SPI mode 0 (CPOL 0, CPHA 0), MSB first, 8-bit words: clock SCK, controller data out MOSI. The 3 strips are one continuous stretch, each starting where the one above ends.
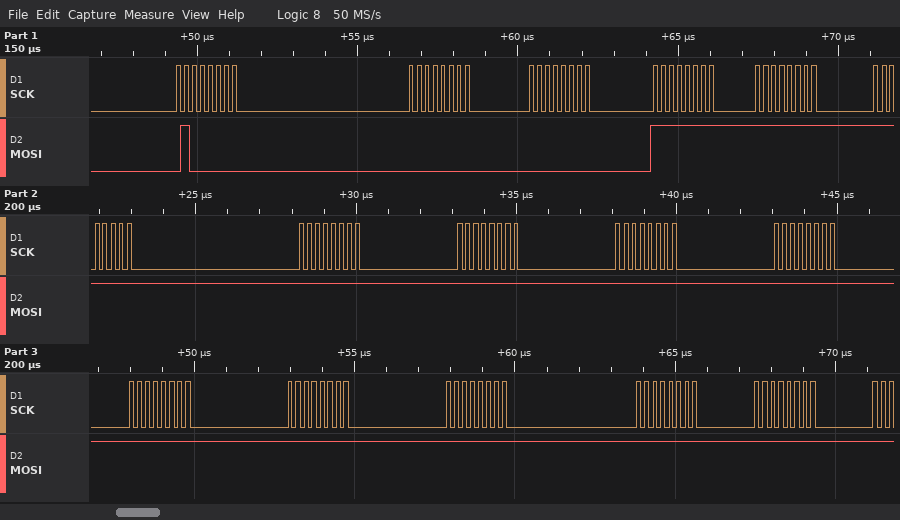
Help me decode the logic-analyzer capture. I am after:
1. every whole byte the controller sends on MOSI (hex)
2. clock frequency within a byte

40 00 00 FF FF FF FF FF FF FF FF FF FF FF FF
4 MHz
